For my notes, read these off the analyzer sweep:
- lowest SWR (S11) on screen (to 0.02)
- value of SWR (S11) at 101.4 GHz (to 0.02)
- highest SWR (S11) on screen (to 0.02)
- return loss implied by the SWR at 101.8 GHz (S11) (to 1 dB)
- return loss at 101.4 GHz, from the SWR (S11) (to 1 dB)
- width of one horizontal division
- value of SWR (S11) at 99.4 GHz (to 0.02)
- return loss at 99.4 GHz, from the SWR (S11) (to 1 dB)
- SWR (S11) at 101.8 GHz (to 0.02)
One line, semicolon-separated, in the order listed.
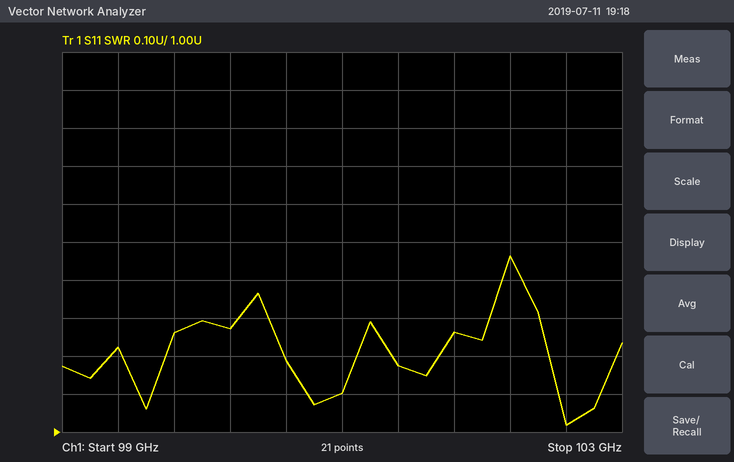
1.02; 1.18; 1.46; 19 dB; 22 dB; 400 MHz; 1.22; 20 dB; 1.26
